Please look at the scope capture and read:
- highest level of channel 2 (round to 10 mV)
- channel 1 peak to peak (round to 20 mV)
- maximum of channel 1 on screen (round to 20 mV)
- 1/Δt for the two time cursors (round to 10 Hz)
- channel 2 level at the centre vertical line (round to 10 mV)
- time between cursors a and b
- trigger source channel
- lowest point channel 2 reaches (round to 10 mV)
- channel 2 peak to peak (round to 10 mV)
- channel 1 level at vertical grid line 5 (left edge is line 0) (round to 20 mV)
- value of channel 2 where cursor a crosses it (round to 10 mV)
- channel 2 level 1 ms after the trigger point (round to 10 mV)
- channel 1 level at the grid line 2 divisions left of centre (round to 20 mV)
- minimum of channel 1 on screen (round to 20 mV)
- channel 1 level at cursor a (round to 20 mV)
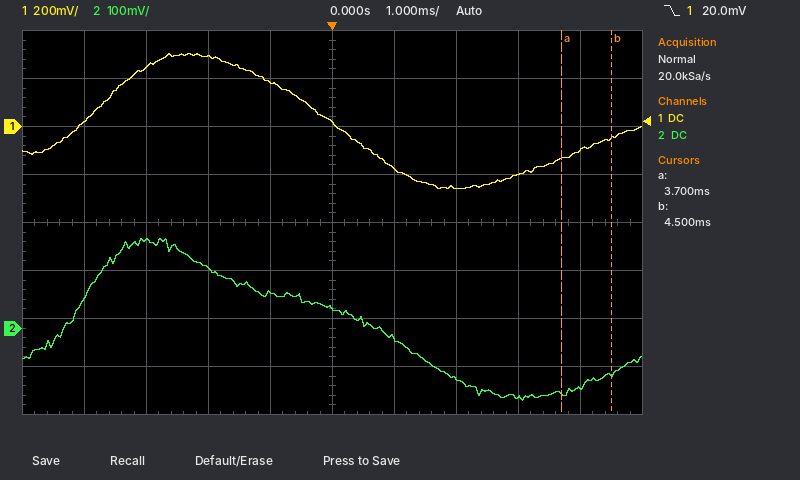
190 mV
560 mV
300 mV
1.25 kHz
40 mV
800 µs
channel 1
-150 mV
340 mV
20 mV
-140 mV
-20 mV
300 mV
-260 mV
-140 mV
